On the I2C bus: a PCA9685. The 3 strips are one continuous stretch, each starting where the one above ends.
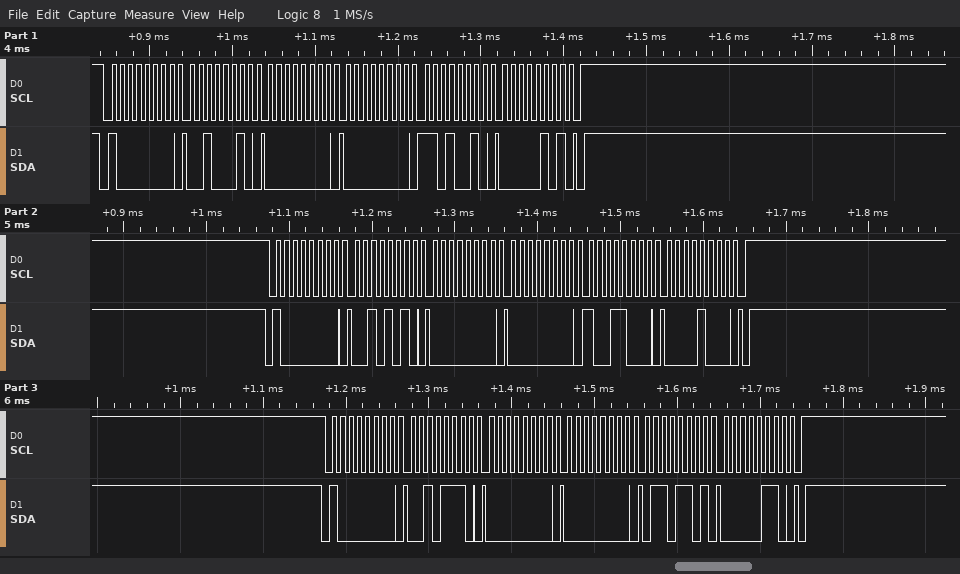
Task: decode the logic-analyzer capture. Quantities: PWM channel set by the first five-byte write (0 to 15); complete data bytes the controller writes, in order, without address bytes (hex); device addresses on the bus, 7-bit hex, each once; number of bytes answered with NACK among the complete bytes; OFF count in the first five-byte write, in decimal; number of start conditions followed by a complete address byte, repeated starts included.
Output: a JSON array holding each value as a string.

["7", "22 00 00 D2 05 2A 00 00 98 08 2E 00 00 6D 06", "0x40", "0", "1490", "3"]
